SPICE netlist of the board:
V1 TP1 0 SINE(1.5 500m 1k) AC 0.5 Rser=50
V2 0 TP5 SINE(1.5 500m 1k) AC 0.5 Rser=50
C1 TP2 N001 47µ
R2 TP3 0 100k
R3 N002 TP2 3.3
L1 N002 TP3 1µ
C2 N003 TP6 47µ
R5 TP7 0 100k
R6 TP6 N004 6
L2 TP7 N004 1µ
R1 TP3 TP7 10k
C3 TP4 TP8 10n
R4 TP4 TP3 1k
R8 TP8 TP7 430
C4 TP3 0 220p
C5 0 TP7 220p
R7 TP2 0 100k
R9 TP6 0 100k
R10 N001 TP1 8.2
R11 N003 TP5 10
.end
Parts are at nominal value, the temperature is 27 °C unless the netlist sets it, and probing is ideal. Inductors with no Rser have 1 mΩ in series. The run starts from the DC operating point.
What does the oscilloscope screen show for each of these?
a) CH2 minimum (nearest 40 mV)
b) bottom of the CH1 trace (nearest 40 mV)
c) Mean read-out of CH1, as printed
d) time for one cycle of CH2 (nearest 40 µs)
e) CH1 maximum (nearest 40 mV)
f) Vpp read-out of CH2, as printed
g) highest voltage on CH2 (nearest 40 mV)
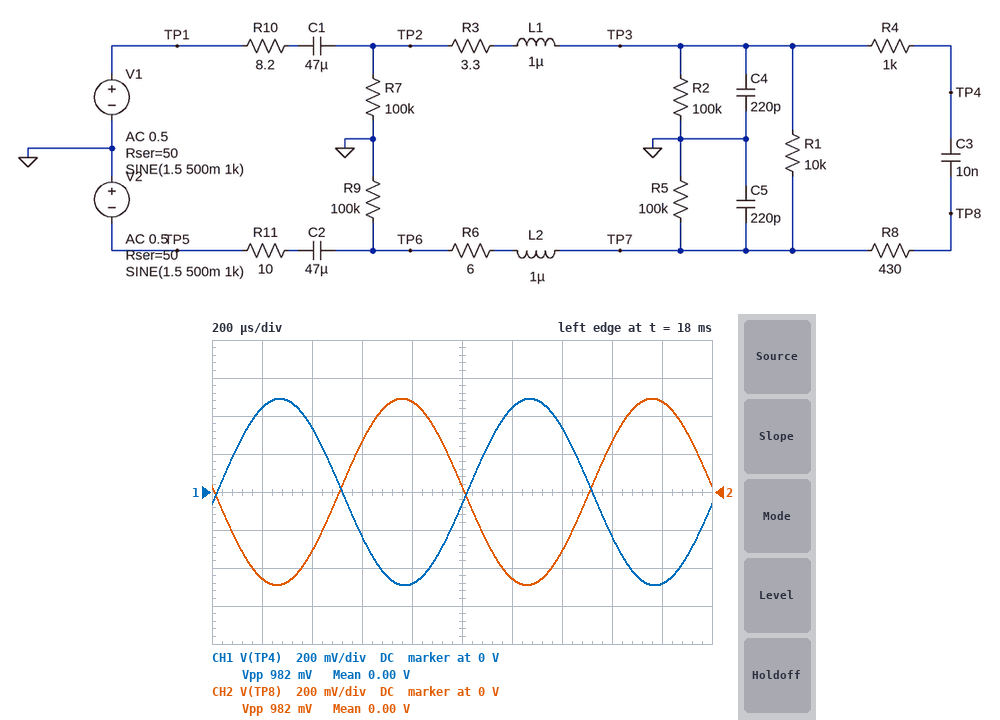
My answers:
-480 mV
-480 mV
0.00 V
1.00 ms
480 mV
982 mV
480 mV
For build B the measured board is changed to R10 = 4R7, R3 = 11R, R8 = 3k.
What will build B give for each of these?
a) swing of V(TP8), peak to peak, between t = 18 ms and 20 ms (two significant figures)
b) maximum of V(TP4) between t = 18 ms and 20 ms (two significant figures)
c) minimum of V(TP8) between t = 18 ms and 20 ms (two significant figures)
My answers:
960 mV
480 mV
-480 mV
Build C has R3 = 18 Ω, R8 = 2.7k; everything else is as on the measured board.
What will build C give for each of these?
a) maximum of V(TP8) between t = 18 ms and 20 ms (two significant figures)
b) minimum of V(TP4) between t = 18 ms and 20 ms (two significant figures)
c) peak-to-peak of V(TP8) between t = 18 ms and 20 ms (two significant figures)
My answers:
480 mV
-480 mV
960 mV
